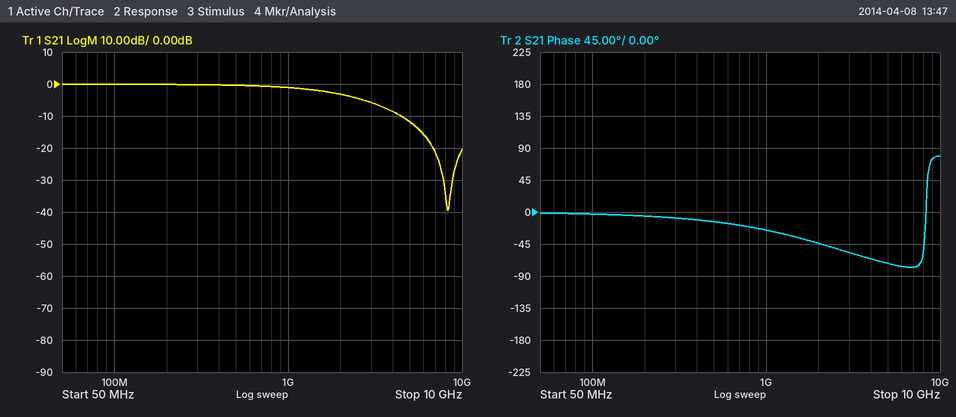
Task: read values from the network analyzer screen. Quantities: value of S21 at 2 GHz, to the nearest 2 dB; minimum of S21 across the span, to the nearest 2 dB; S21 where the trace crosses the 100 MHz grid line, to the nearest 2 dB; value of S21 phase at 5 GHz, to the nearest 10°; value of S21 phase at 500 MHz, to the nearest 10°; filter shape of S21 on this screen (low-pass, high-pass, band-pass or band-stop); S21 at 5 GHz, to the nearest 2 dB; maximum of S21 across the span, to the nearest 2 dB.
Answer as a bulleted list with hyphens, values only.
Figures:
- -4 dB
- -40 dB
- 0 dB
- -70°
- -10°
- low-pass
- -12 dB
- 0 dB
